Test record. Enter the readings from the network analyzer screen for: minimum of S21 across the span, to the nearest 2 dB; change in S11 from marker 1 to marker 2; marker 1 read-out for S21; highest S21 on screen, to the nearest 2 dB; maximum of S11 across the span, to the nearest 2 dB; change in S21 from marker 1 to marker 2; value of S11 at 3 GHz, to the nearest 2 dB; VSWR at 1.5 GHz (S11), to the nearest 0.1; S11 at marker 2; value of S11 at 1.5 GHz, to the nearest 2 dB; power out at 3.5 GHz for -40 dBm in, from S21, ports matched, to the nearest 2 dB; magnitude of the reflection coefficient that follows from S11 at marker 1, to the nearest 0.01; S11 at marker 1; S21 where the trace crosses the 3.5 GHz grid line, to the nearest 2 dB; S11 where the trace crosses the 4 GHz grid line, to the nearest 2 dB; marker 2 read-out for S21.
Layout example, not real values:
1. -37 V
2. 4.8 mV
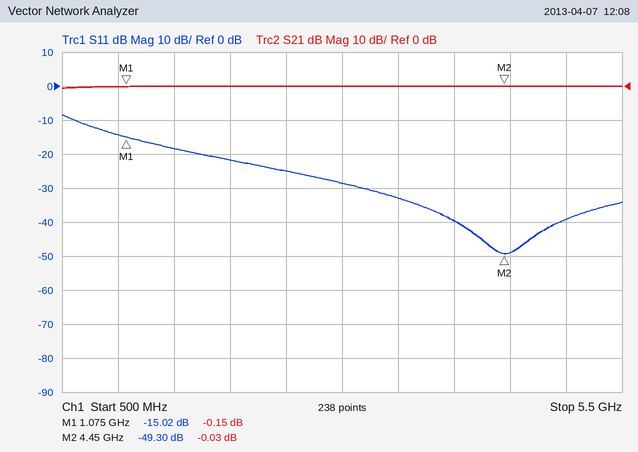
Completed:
1. 0 dB
2. -34.28 dB
3. -0.15 dB
4. 0 dB
5. -8 dB
6. 0.12 dB
7. -28 dB
8. 1.3
9. -49.30 dB
10. -18 dB
11. -40 dBm
12. 0.18
13. -15.02 dB
14. 0 dB
15. -40 dB
16. -0.03 dB
